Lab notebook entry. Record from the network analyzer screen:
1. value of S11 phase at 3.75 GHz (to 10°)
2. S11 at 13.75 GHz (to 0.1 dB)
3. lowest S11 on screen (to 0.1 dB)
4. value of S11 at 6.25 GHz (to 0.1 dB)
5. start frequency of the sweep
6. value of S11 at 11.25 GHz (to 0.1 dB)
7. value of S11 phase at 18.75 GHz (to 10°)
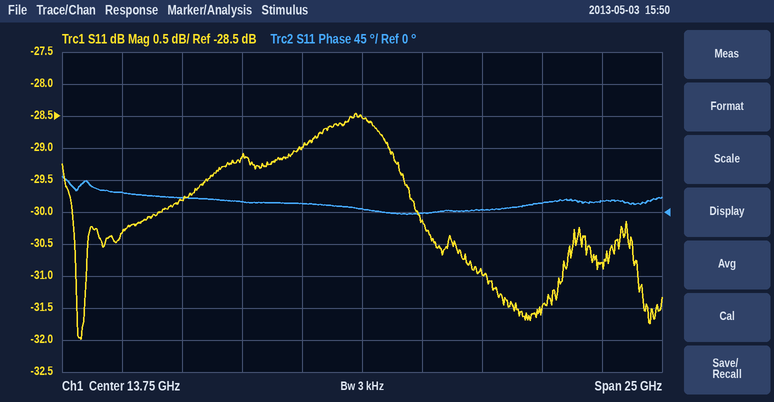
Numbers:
30°
-28.5 dB
-32.0 dB
-29.8 dB
1.25 GHz
-29.0 dB
0°
